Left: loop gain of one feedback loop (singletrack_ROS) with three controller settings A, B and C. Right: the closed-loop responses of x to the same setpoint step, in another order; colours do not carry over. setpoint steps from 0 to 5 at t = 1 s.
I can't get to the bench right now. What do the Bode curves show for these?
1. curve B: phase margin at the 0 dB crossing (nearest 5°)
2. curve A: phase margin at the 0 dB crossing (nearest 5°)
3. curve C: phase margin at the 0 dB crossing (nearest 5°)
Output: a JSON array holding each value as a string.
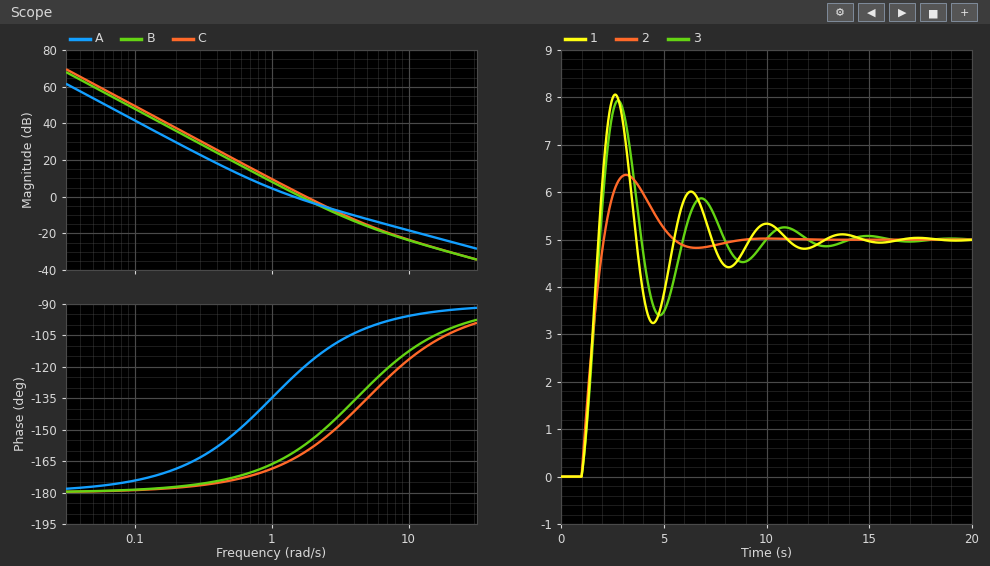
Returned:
["20°", "55°", "20°"]
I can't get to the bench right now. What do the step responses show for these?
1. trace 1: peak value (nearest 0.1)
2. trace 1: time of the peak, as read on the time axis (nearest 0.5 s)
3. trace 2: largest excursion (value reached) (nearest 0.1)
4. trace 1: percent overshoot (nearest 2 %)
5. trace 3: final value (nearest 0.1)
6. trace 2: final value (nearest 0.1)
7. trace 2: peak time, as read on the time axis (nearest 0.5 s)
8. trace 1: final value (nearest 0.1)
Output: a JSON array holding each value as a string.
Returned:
["8.1", "2.5 s", "6.4", "62 %", "5.0", "5.0", "3.0 s", "5.0"]
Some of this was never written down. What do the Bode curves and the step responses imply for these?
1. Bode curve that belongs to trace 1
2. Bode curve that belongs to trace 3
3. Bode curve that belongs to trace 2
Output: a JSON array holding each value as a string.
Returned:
["C", "B", "A"]
